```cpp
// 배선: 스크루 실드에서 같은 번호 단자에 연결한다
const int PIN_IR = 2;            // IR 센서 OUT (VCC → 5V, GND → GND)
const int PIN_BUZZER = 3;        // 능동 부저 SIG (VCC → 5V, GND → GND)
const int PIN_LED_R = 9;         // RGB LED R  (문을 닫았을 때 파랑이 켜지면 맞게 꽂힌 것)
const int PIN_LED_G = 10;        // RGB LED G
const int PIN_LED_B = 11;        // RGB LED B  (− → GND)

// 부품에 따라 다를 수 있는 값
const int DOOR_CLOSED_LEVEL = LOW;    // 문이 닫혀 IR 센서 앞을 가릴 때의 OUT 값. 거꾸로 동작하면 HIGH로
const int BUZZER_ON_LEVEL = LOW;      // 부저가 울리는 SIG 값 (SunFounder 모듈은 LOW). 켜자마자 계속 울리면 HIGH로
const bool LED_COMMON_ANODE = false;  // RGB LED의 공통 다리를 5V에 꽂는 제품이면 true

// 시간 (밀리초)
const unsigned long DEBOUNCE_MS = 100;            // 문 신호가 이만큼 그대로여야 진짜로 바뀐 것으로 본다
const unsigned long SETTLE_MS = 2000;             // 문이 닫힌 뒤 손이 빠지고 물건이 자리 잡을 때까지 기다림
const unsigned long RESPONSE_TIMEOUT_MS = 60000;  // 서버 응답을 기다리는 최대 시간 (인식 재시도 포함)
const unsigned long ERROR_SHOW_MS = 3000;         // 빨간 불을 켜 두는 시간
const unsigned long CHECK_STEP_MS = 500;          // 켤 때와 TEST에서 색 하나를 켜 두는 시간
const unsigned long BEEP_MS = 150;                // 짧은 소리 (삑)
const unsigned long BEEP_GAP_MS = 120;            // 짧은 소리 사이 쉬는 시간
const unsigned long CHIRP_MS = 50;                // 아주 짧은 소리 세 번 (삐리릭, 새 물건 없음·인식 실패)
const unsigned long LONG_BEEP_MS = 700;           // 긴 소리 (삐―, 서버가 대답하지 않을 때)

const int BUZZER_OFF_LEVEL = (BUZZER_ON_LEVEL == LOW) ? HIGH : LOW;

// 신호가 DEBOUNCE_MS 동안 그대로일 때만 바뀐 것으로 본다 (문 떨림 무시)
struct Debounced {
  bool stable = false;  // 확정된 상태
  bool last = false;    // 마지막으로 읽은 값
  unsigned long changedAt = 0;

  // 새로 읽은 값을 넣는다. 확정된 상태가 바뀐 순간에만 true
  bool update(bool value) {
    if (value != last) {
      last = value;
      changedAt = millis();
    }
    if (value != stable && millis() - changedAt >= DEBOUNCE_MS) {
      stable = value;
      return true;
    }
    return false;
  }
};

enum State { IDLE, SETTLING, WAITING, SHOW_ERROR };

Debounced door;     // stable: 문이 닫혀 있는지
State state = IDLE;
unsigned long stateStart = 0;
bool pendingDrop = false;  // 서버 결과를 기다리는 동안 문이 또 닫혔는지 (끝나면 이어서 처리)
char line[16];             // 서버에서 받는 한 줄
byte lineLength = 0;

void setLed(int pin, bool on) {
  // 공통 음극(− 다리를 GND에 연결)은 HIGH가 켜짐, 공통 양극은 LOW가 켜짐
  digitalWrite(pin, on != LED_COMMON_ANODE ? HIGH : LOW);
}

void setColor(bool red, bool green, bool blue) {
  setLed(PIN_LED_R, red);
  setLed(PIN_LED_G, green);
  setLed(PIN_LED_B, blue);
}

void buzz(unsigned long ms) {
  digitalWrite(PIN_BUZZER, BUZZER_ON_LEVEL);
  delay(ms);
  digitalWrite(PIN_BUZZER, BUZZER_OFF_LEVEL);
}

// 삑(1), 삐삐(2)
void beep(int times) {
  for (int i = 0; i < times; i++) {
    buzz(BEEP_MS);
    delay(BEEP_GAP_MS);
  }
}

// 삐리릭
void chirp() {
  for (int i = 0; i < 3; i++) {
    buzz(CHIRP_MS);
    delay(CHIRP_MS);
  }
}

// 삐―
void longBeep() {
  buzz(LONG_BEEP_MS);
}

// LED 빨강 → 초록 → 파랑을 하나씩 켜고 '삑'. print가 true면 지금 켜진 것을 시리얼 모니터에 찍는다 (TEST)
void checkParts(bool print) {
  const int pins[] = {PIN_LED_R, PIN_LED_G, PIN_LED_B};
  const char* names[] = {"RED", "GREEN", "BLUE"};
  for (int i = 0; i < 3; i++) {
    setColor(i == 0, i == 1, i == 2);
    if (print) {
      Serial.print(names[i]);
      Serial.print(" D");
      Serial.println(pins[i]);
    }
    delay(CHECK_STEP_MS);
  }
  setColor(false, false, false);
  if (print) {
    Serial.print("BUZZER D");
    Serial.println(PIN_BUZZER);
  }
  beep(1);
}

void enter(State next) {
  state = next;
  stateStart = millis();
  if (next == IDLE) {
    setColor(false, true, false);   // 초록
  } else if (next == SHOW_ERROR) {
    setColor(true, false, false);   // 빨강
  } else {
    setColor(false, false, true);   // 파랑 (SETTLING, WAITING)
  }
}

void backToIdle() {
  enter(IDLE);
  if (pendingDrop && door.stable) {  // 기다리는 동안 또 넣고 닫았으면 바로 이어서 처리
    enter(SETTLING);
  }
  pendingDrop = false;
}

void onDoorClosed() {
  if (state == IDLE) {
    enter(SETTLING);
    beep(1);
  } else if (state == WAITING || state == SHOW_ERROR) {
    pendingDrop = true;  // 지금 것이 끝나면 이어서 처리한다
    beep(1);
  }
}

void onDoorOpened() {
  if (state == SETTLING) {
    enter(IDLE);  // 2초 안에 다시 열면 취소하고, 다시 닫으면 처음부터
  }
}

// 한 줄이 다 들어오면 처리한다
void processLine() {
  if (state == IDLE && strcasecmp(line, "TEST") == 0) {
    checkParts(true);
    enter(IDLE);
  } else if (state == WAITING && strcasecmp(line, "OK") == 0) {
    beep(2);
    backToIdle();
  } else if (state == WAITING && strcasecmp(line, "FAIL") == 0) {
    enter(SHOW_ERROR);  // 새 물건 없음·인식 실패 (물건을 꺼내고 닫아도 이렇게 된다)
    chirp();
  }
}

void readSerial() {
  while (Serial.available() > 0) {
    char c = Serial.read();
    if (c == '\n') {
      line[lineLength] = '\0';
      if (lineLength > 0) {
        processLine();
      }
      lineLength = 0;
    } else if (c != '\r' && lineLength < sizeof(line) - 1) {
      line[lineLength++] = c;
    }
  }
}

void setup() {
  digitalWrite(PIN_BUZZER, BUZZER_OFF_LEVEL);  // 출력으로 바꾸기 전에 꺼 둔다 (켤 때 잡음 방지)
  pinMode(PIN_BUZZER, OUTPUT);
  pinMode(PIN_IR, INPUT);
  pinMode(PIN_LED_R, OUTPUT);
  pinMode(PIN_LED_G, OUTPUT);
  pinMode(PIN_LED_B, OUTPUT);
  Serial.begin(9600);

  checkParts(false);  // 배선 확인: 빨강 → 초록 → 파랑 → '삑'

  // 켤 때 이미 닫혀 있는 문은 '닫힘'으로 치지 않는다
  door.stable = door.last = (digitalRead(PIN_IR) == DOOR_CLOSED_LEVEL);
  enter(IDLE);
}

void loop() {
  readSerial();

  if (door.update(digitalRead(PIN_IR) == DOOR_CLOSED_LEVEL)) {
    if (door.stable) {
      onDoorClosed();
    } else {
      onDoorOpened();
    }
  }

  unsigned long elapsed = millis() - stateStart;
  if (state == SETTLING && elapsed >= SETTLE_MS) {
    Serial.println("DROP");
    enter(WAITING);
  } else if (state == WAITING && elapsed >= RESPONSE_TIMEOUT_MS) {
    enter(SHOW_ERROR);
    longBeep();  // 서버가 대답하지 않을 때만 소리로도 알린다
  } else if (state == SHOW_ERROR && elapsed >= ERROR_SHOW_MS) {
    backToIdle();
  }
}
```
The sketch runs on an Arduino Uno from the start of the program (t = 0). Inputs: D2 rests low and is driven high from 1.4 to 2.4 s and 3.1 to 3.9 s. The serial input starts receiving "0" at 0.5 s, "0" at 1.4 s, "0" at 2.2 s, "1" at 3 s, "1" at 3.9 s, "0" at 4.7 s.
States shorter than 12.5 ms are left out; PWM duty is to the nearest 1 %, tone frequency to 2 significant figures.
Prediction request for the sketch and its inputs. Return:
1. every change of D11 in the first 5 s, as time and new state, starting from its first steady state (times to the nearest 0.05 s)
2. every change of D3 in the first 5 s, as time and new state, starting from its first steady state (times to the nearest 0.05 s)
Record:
0 s low; 1 s high; 1.5 s low; 2.5 s high; 3.2 s low; 4 s high
0 s high; 1.5 s low; 1.65 s high; 2.5 s low; 2.65 s high; 4 s low; 4.15 s high
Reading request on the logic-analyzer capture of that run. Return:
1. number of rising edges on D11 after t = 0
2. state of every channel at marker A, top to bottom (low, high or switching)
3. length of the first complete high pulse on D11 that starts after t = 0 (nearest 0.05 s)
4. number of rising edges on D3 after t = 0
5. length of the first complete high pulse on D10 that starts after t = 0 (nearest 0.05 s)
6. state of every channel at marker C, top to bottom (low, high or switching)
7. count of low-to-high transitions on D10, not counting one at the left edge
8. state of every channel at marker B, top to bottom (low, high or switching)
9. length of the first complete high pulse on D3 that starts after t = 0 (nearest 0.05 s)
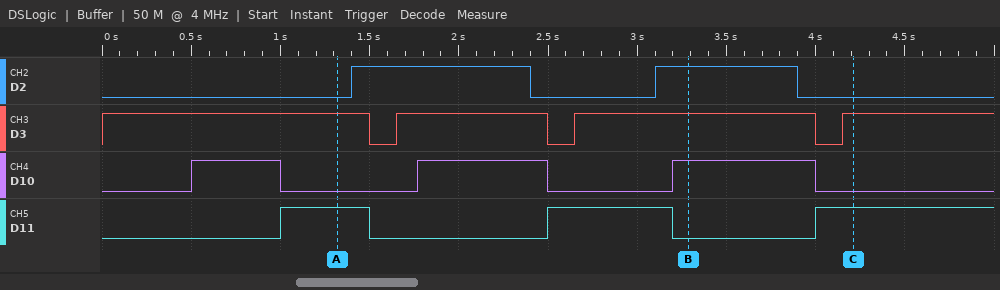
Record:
3
D2 low, D3 high, D10 low, D11 high
0.50 s
3
0.50 s
D2 low, D3 high, D10 low, D11 high
3
D2 high, D3 high, D10 high, D11 low
0.85 s
